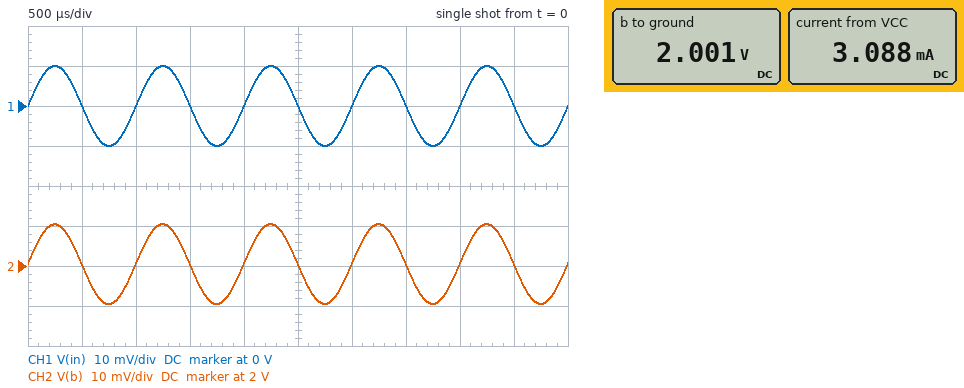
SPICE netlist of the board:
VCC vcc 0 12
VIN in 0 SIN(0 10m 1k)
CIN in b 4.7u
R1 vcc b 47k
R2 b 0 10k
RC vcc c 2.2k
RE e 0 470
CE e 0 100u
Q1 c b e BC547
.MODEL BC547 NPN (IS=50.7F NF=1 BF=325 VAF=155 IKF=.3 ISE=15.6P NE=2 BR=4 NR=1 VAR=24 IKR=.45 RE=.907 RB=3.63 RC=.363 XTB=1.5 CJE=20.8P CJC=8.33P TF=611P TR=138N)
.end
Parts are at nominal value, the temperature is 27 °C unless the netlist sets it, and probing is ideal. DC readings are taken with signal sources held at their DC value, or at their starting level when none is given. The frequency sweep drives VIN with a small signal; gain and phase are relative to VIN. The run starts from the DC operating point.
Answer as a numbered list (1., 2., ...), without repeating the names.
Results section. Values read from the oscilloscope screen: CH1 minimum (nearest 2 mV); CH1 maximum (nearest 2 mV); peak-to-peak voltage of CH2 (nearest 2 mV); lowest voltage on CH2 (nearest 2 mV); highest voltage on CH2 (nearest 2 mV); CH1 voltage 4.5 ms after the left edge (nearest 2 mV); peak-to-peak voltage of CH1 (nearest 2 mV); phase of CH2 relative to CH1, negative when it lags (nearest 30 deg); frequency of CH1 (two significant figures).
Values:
1. -10 mV
2. 10 mV
3. 20 mV
4. 1.990 V
5. 2.010 V
6. 0 V
7. 20 mV
8. 0 deg
9. 1.0 kHz
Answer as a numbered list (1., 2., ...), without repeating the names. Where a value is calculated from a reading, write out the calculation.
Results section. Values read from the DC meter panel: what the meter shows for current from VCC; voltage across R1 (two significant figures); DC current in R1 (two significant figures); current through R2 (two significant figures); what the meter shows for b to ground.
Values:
1. 3.088 mA
2. 12 V - 2.001 V = 10 V
3. (12 V - 2.001 V) / 47 kΩ = 210 µA
4. (2.001 V) / 10 kΩ = 200 µA
5. 2.001 V
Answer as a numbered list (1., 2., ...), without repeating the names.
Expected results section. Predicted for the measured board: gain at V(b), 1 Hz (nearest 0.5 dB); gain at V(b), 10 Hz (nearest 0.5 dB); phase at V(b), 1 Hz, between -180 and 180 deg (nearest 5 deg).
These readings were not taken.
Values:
1. -13.0 dB
2. -1.5 dB
3. 75 deg
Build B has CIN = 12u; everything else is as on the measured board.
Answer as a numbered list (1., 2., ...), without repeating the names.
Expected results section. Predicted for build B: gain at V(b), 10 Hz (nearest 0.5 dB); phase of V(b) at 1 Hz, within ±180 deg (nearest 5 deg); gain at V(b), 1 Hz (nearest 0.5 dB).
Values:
1. -0.5 dB
2. 60 deg
3. -6.0 dB
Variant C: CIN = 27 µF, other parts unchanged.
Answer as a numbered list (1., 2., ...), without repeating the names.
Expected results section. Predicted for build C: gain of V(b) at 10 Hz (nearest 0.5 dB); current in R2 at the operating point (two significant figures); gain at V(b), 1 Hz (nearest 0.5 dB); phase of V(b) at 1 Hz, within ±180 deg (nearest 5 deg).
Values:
1. 0 dB
2. 200 µA
3. -2.0 dB
4. 35 deg
